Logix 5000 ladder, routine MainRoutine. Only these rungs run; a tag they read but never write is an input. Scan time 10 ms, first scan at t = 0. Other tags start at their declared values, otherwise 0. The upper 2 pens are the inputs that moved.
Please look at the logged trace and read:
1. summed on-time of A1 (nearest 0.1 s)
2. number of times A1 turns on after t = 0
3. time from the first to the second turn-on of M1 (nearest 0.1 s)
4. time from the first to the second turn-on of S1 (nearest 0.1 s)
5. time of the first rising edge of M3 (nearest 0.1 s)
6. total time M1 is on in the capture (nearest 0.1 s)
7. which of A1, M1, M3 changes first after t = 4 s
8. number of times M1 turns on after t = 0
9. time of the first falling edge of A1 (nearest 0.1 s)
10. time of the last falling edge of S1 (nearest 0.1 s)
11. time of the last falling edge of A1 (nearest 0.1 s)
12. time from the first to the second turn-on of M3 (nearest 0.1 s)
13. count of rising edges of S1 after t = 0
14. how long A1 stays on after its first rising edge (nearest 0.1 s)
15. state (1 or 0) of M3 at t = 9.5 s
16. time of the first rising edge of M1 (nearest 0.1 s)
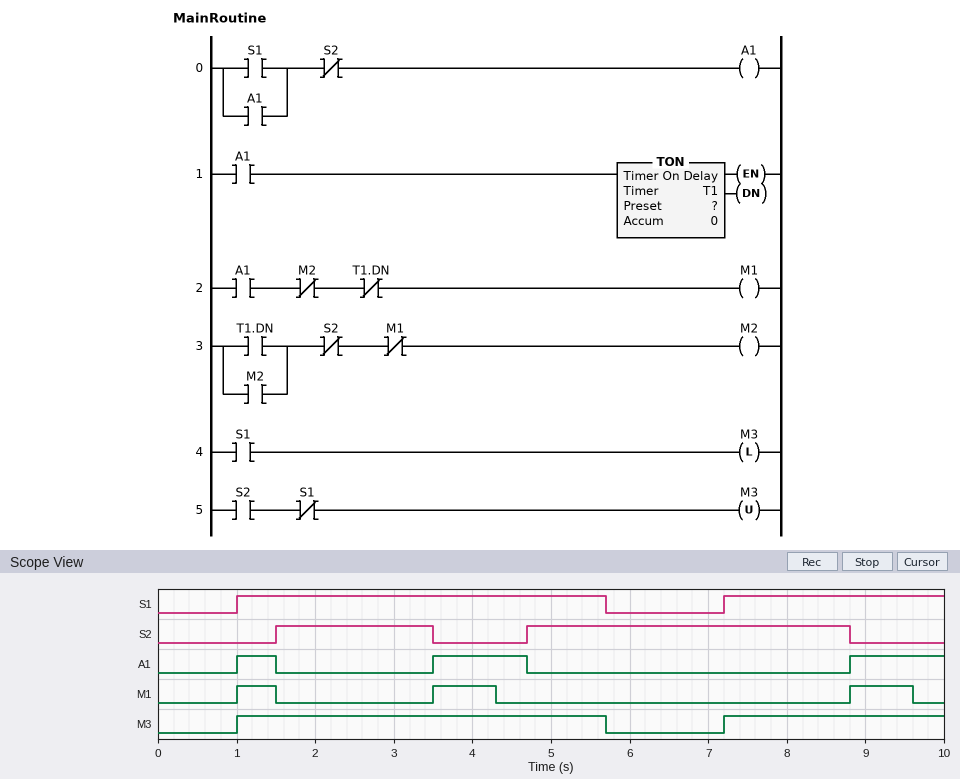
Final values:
2.9 s
3
2.5 s
6.2 s
1.0 s
2.1 s
M1
3
1.5 s
5.7 s
4.7 s
6.2 s
2
0.5 s
1
1.0 s
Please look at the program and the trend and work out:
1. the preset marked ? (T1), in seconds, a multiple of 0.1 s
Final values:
0.8 s
